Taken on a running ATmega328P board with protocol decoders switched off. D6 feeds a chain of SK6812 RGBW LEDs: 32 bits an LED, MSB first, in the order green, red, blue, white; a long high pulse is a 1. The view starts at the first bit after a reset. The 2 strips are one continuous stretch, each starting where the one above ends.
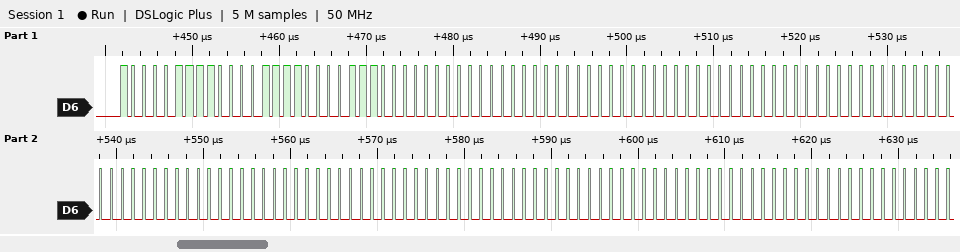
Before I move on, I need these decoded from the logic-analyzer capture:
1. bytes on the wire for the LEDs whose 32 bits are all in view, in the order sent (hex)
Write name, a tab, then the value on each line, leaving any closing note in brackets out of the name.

bytes on the wire for the LEDs whose 32 bits are all in view, in the order sent	87 87 87 00 00 00 00 00 00 00 00 00 00 00 00 00
